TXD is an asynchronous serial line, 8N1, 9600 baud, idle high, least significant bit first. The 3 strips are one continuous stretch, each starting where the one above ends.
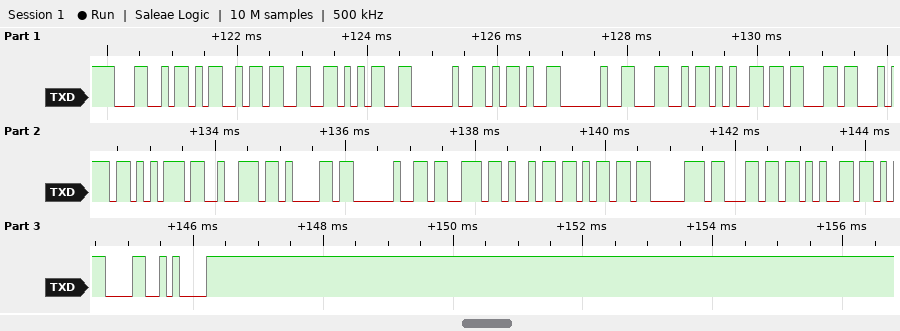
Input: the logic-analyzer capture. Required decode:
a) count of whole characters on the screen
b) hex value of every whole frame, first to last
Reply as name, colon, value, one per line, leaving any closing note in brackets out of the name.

count of whole characters on the screen: 23
hex value of every whole frame, first to last: 0x4C 0x4D 0x33 0x35 0x20 0x2D 0x20 0x4C 0x65 0x63 0x74 0x75 0x72 0x61 0x20 0x73 0x69 0x6D 0x70 0x6C 0x65 0x0D 0x0A
